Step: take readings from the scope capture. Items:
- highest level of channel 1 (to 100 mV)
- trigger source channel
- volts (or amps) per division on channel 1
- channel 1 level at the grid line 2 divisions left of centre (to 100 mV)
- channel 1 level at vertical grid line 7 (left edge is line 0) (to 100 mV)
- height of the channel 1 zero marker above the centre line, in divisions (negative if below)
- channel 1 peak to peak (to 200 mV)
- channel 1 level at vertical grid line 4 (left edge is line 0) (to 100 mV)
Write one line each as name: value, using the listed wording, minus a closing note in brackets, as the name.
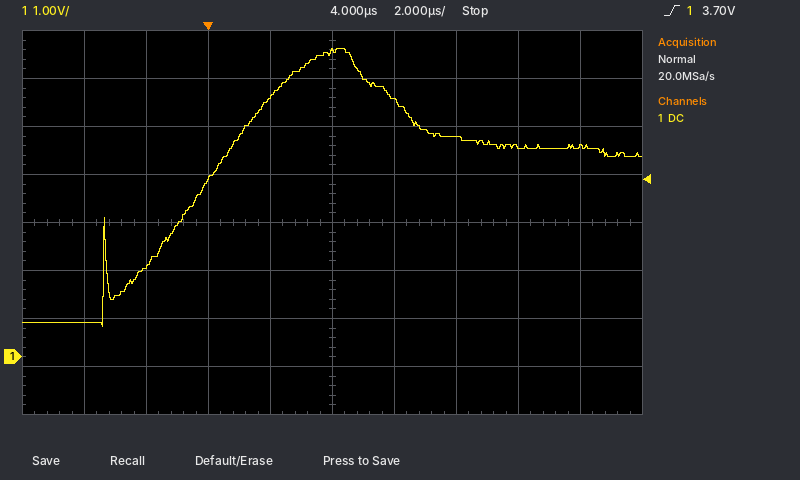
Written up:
highest level of channel 1: 6.4 V
trigger source channel: channel 1
volts (or amps) per division on channel 1: 1 V
channel 1 level at the grid line 2 divisions left of centre: 3.7 V
channel 1 level at vertical grid line 7 (left edge is line 0): 4.6 V
height of the channel 1 zero marker above the centre line, in divisions: -2.8 div
channel 1 peak to peak: 5.8 V
channel 1 level at vertical grid line 4 (left edge is line 0): 5.4 V
